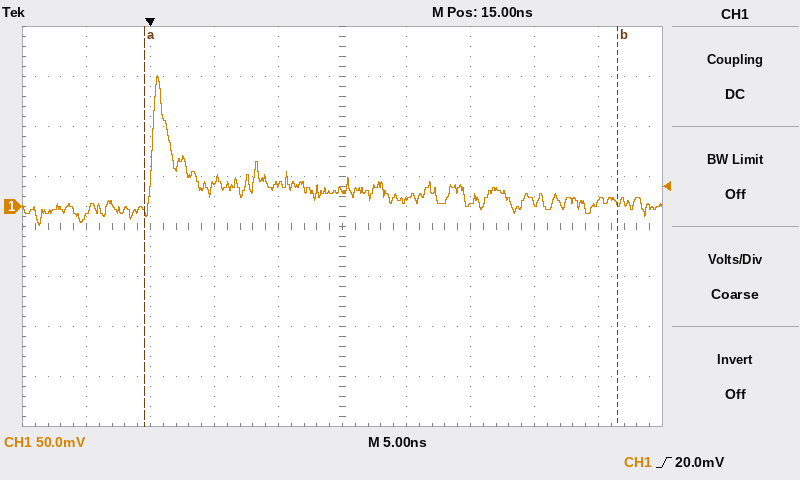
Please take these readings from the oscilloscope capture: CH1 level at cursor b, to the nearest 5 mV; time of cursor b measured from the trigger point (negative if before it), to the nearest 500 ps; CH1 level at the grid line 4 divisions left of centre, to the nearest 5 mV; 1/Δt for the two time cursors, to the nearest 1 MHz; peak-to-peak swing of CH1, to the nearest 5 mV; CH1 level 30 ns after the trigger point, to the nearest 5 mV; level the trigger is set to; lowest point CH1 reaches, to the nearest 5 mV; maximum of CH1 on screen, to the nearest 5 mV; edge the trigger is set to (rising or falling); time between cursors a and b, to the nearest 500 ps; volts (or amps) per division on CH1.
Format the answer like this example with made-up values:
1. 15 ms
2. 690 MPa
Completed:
1. 5 mV
2. +36.5 ns
3. -10 mV
4. 27 MHz
5. 150 mV
6. 5 mV
7. 20.0 mV
8. -20 mV
9. 130 mV
10. rising
11. 37.0 ns
12. 50 mV
